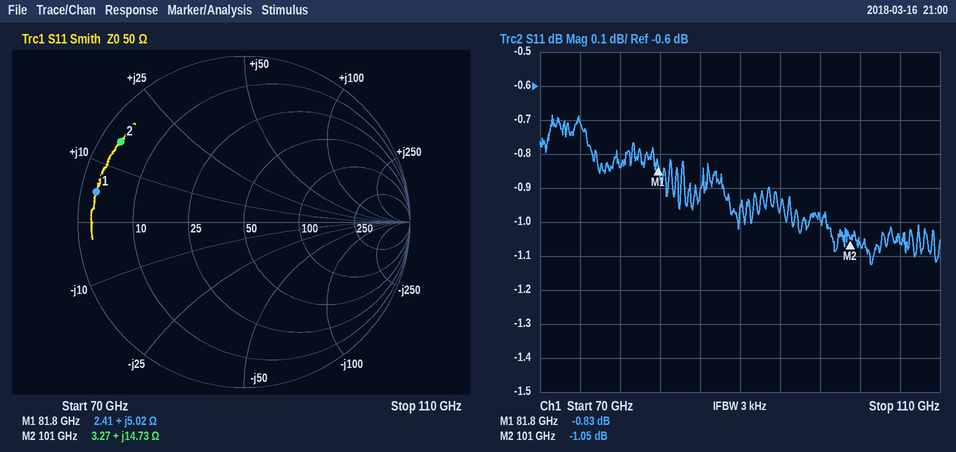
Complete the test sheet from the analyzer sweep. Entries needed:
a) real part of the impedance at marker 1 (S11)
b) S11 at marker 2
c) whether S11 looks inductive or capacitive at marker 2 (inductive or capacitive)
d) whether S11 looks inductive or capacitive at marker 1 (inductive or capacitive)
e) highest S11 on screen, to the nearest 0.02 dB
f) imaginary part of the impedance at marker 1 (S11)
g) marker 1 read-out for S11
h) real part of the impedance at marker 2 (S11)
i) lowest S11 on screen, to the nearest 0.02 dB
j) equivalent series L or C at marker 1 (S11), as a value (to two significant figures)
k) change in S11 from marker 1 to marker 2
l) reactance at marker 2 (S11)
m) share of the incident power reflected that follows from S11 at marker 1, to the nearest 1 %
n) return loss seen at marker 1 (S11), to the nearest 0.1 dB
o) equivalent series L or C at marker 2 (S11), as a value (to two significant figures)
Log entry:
2.41 Ω
-1.05 dB
inductive
inductive
-0.68 dB
+5.02 Ω
-0.83 dB
3.27 Ω
-1.12 dB
9.8 pH
-0.22 dB
+14.73 Ω
83 %
0.8 dB
23 pH
